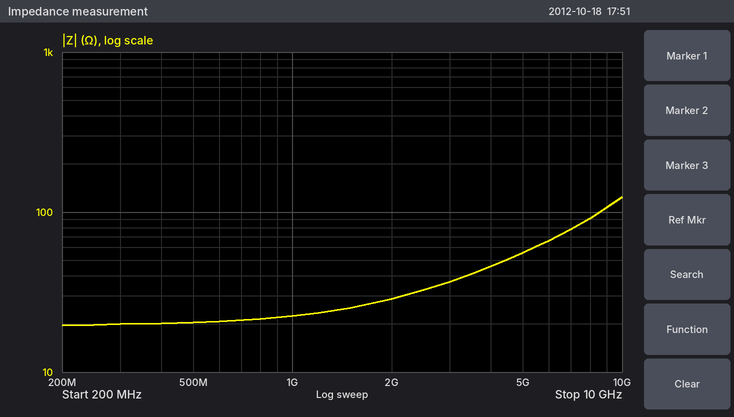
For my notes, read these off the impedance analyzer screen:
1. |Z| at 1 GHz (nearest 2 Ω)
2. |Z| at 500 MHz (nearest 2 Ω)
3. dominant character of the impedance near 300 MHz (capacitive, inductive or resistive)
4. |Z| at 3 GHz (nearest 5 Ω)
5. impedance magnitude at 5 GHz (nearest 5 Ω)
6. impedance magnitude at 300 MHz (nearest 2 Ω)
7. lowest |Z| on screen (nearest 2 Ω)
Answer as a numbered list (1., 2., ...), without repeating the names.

1. 22 Ω
2. 20 Ω
3. resistive
4. 35 Ω
5. 55 Ω
6. 20 Ω
7. 20 Ω
